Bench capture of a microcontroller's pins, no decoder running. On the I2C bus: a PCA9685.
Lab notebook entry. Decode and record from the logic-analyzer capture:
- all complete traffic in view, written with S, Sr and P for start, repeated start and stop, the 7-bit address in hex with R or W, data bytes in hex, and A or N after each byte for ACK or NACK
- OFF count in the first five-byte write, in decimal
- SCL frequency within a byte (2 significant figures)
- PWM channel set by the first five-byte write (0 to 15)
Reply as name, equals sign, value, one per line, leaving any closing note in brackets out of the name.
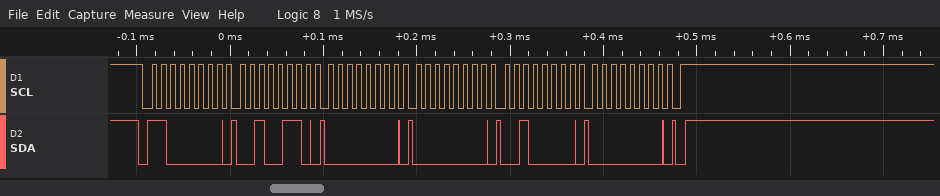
all complete traffic in view, written with S, Sr and P for start, repeated start and stop, the 7-bit address in hex with R or W, data bytes in hex, and A or N after each byte for ACK or NACK = S 60W A 26 A 00 A 00 A 20 A 00 A P
OFF count in the first five-byte write, in decimal = 32
SCL frequency within a byte = 100 kHz
PWM channel set by the first five-byte write = 8
